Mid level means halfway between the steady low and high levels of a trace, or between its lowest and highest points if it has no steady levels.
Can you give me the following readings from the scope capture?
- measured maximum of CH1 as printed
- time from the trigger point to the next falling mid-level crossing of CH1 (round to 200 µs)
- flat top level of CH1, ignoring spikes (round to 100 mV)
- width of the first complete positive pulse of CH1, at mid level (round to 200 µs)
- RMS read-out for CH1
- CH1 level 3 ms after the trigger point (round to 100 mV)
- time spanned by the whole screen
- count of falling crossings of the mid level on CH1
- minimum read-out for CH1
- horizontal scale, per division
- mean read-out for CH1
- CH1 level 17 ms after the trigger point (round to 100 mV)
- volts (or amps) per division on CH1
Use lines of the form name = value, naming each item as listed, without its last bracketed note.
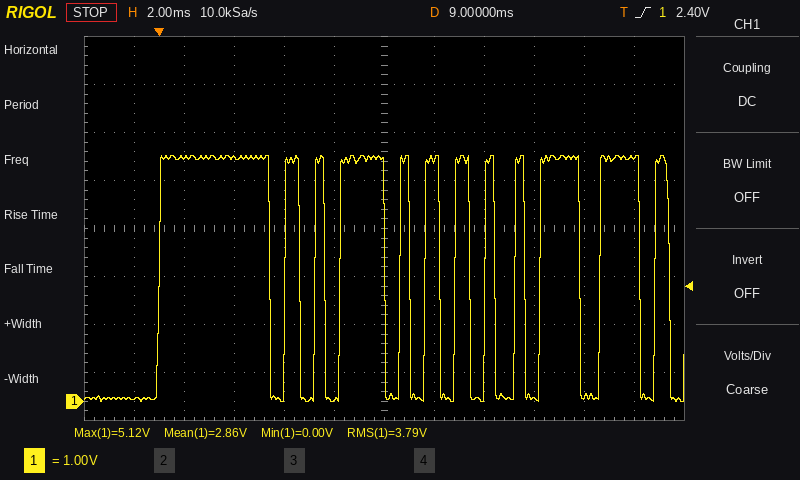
measured maximum of CH1 as printed = 5.12 V
time from the trigger point to the next falling mid-level crossing of CH1 = 4.4 ms
flat top level of CH1, ignoring spikes = 5.1 V
width of the first complete positive pulse of CH1, at mid level = 4.4 ms
RMS read-out for CH1 = 3.79 V
CH1 level 3 ms after the trigger point = 5.1 V
time spanned by the whole screen = 24 ms
count of falling crossings of the mid level on CH1 = 12
minimum read-out for CH1 = 0.00 V
horizontal scale, per division = 2 ms
mean read-out for CH1 = 2.86 V
CH1 level 17 ms after the trigger point = 100 mV
volts (or amps) per division on CH1 = 1 V
